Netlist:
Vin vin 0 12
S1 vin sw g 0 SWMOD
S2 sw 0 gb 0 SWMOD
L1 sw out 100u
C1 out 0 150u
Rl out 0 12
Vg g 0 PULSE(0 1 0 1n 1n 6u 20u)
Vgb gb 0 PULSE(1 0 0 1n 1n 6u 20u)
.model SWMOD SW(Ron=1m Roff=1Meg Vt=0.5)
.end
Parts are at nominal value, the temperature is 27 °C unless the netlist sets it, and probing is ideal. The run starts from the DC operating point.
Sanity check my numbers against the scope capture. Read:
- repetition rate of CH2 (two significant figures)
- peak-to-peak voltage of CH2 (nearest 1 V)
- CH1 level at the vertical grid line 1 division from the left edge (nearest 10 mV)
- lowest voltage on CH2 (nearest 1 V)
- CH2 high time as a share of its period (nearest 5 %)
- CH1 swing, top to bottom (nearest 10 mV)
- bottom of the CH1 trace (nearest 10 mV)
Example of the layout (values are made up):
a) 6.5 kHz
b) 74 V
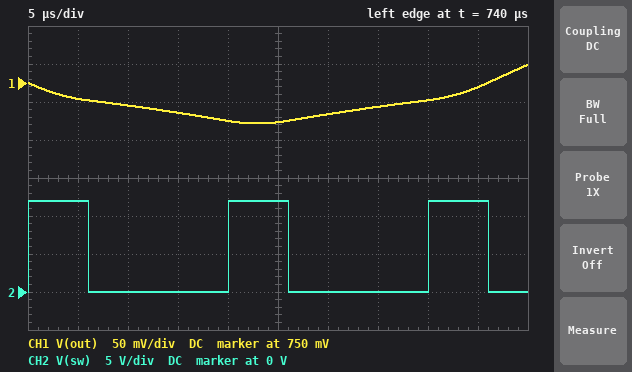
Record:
a) 50 kHz
b) 12 V
c) 730 mV
d) 0 V
e) 30 %
f) 80 mV
g) 700 mV
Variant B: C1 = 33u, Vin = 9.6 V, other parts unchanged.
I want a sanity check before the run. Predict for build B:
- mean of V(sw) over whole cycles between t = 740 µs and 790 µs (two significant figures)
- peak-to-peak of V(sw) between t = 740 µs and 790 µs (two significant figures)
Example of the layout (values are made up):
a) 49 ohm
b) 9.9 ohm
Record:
a) 2.9 V
b) 9.6 V
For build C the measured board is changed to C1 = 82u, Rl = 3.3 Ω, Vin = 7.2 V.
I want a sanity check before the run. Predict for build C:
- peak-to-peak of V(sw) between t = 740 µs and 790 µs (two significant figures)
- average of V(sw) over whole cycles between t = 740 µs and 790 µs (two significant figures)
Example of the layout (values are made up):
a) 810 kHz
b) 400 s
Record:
a) 7.2 V
b) 2.2 V
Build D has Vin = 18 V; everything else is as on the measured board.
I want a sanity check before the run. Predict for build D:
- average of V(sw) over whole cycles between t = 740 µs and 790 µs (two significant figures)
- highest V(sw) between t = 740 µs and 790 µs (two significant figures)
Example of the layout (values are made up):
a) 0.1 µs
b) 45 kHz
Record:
a) 5.4 V
b) 18 V
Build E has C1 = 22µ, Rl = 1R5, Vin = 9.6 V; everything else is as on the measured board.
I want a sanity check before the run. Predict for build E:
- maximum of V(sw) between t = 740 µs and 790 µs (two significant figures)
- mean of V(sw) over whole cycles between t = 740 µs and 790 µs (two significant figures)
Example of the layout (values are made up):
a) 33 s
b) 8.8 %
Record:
a) 9.6 V
b) 2.9 V
